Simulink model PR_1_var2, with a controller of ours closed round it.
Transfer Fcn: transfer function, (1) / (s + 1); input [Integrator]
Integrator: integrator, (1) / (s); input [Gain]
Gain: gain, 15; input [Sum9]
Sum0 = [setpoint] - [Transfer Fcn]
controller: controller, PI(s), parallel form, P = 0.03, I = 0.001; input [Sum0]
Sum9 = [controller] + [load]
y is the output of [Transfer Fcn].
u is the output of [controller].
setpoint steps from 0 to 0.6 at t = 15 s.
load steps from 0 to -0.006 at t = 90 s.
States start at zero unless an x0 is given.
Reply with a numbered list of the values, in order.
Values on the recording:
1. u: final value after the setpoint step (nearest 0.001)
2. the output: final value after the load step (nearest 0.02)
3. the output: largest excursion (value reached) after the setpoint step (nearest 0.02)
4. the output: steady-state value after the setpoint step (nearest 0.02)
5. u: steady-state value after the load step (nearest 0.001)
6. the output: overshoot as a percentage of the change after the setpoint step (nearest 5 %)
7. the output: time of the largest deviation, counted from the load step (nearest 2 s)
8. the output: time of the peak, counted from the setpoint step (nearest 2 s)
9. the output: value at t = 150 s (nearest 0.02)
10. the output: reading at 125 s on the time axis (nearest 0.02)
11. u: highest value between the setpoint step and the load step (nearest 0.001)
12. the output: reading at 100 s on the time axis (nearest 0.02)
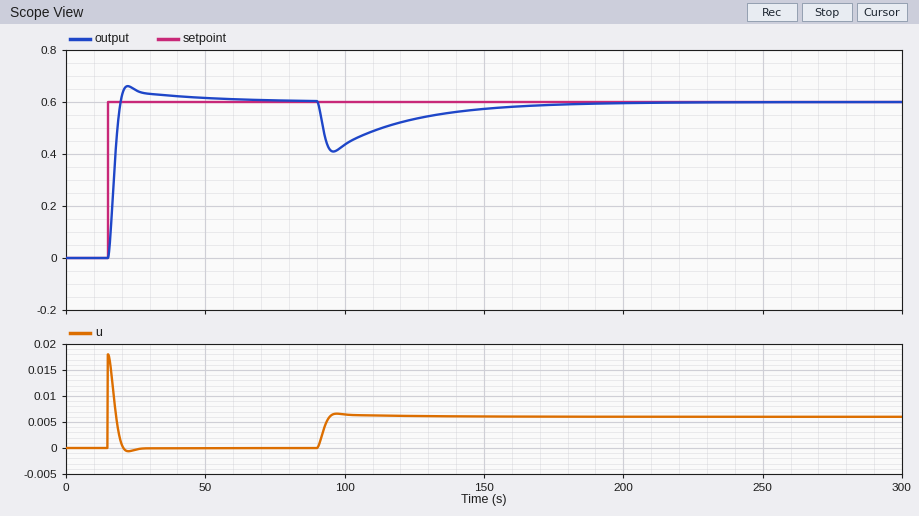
1. 0.000
2. 0.60
3. 0.66
4. 0.60
5. 0.006
6. 10 %
7. 6 s
8. 8 s
9. 0.58
10. 0.54
11. 0.018
12. 0.44
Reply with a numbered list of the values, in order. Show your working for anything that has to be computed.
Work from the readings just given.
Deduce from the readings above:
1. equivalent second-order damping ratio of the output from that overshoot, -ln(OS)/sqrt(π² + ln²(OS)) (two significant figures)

1. ln(0.1) = -2.303; 2.303 / sqrt(9.870 + 5.302) = 0.59
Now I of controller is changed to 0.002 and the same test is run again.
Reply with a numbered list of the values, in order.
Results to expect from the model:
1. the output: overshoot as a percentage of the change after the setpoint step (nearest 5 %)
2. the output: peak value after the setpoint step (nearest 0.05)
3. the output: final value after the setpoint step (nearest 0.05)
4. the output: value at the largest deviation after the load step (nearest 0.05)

1. 15 %
2. 0.70
3. 0.60
4. 0.40
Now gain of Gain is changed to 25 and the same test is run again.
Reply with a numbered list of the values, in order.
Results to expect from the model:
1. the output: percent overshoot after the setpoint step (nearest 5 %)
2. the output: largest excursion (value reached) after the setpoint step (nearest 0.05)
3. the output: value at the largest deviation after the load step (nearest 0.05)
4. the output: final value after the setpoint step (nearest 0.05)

1. 15 %
2. 0.70
3. 0.40
4. 0.60
